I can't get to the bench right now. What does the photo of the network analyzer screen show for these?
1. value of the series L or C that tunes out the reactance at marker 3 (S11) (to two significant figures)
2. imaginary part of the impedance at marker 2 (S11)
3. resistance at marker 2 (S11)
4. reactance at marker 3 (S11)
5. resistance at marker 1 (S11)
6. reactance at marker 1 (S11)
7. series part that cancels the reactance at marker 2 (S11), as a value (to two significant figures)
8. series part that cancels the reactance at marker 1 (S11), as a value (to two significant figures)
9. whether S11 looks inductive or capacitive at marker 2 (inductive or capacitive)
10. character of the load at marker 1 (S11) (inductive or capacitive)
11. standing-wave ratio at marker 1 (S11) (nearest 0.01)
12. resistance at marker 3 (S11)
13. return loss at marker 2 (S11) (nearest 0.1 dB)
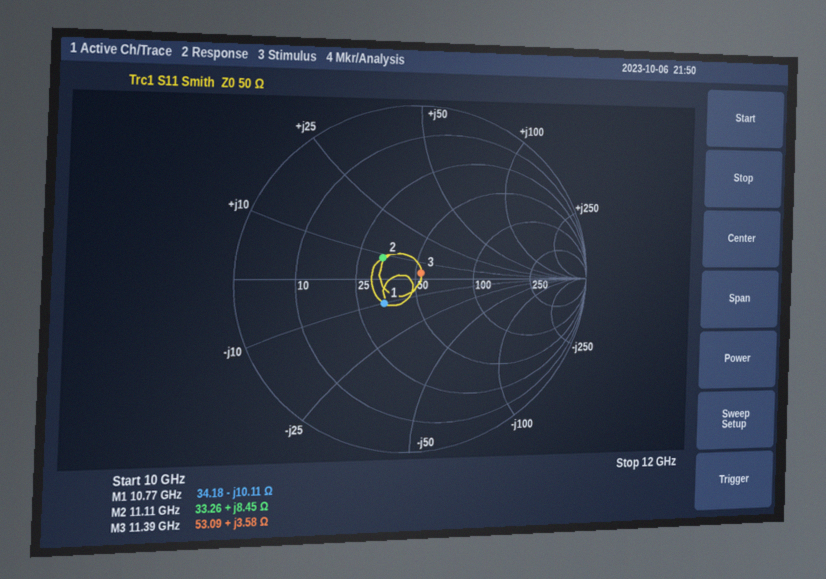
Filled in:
3.9 pF
+8.45 Ω
33.26 Ω
+3.58 Ω
34.18 Ω
-10.11 Ω
1.7 pF
150 pH
inductive
capacitive
1.57
53.09 Ω
13.0 dB
